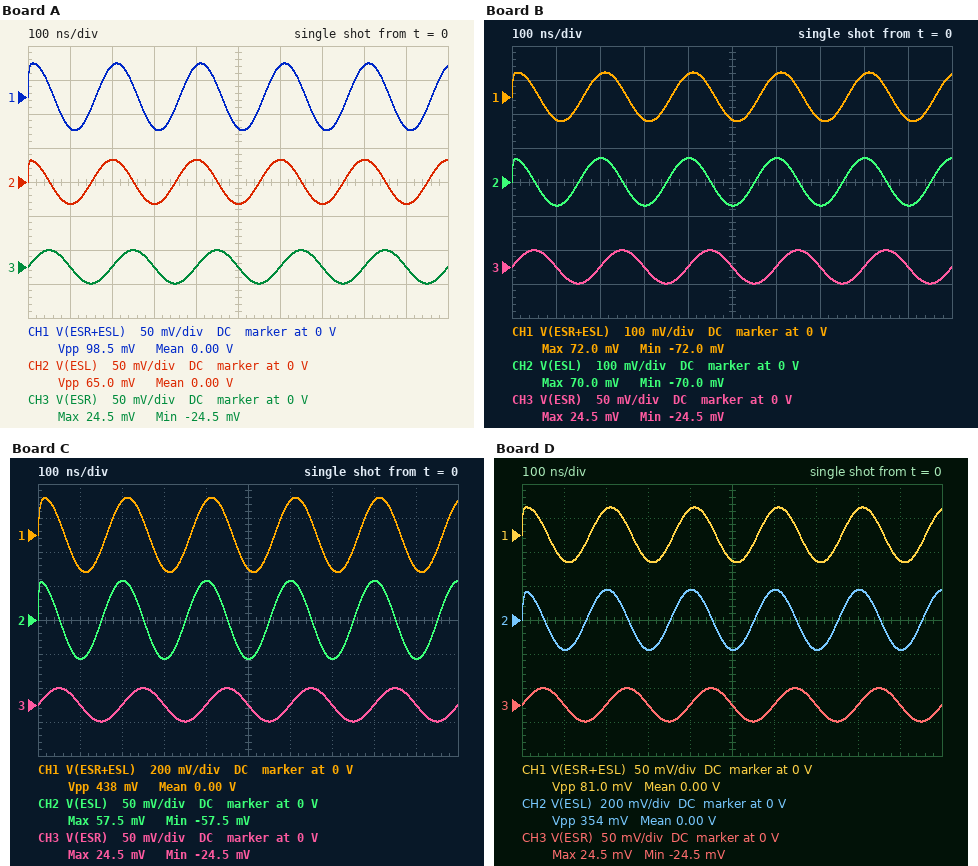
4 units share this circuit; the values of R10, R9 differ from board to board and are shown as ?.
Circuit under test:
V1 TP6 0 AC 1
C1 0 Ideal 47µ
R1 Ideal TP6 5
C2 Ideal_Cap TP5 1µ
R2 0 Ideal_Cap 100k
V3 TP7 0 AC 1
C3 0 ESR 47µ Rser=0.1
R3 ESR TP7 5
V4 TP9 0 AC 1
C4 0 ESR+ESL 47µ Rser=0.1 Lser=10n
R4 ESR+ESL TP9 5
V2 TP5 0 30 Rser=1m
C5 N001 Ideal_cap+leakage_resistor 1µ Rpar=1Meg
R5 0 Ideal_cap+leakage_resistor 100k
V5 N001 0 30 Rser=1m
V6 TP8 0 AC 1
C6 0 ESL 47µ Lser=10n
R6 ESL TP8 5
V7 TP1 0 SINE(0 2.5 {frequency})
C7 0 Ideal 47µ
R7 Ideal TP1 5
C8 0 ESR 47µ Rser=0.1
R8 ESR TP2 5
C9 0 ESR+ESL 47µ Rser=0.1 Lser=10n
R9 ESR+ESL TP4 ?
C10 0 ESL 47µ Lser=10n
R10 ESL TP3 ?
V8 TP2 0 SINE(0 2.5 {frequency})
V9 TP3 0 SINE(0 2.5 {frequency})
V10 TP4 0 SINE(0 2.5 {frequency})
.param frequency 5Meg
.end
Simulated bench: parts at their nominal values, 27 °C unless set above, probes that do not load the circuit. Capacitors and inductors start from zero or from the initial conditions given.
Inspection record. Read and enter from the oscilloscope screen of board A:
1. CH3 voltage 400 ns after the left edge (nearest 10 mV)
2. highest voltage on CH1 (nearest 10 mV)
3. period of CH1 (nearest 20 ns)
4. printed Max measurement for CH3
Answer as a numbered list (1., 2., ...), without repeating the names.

1. 0 V
2. 50 mV
3. 200 ns
4. 24.5 mV
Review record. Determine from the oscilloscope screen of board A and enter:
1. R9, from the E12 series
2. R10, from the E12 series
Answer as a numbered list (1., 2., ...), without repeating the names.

1. 8.2 Ω
2. 12 Ω
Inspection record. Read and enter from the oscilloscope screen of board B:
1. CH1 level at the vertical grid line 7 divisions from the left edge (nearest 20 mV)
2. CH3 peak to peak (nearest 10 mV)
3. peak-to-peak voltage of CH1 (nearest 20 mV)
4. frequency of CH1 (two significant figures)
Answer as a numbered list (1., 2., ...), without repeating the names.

1. -60 mV
2. 50 mV
3. 140 mV
4. 5.0 MHz
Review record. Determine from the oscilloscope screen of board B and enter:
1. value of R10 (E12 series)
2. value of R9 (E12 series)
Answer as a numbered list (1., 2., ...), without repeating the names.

1. 5.6 Ω
2. 5.6 Ω
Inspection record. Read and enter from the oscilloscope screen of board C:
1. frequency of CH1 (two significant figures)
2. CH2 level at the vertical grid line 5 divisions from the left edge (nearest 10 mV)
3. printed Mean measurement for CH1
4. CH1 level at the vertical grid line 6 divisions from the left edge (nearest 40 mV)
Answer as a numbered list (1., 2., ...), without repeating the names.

1. 5.0 MHz
2. -60 mV
3. 0.00 V
4. 200 mV
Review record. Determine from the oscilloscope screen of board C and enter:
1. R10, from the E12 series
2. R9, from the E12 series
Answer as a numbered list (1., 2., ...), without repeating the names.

1. 6.8 Ω
2. 1.8 Ω
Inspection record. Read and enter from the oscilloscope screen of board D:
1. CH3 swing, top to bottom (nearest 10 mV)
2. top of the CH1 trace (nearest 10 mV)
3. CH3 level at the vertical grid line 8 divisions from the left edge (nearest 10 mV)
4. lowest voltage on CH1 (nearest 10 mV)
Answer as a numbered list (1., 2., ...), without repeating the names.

1. 50 mV
2. 40 mV
3. 0 V
4. -40 mV
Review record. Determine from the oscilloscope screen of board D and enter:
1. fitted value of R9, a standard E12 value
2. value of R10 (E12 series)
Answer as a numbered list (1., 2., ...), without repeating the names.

1. 10 Ω
2. 2.2 Ω
